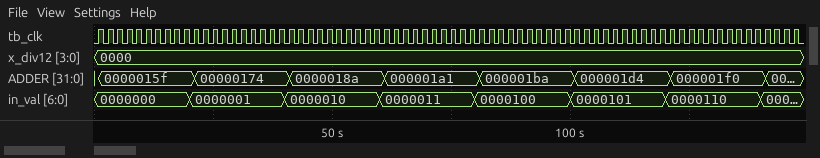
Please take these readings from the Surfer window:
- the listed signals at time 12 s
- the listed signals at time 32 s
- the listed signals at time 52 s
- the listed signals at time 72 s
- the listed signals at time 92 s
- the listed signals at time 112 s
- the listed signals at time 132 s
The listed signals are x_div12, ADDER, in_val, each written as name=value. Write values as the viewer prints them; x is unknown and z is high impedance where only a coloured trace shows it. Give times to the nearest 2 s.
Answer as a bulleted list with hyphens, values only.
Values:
- x_div12=0000, ADDER=0000015f, in_val=0000000
- x_div12=0000, ADDER=00000174, in_val=0000001
- x_div12=0000, ADDER=0000018a, in_val=0000010
- x_div12=0000, ADDER=000001a1, in_val=0000011
- x_div12=0000, ADDER=000001ba, in_val=0000100
- x_div12=0000, ADDER=000001d4, in_val=0000101
- x_div12=0000, ADDER=000001f0, in_val=0000110
